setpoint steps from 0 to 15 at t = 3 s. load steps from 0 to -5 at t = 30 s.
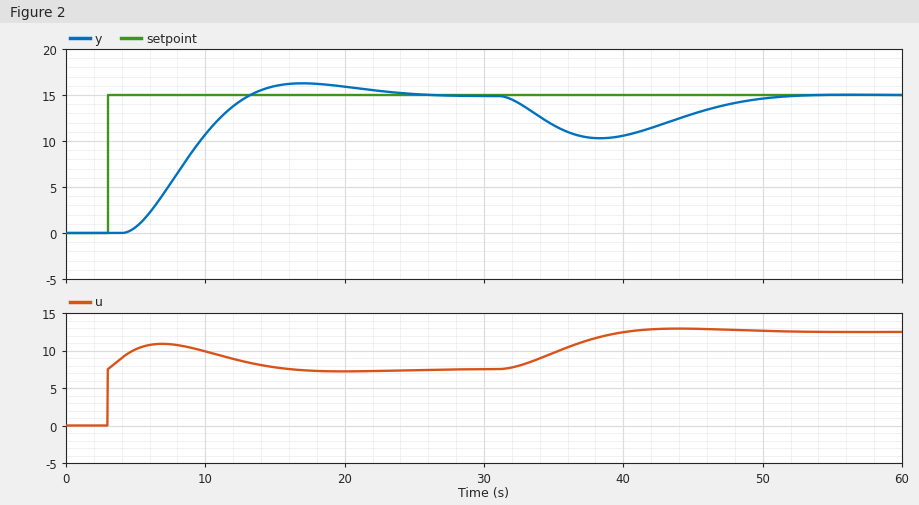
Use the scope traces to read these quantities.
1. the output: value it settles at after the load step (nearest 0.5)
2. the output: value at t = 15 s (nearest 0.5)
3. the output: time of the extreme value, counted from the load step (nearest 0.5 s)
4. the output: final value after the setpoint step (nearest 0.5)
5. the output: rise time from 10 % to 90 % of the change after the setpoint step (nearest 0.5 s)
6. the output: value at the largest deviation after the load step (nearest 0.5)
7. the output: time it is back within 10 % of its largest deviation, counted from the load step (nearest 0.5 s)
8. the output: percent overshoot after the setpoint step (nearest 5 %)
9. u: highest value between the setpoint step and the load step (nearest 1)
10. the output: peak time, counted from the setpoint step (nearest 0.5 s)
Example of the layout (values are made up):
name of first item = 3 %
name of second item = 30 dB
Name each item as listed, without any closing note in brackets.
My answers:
the output: value it settles at after the load step = 15.0
the output: value at t = 15 s = 16.0
the output: time of the extreme value, counted from the load step = 8.5 s
the output: final value after the setpoint step = 15.0
the output: rise time from 10 % to 90 % of the change after the setpoint step = 6.0 s
the output: value at the largest deviation after the load step = 10.5
the output: time it is back within 10 % of its largest deviation, counted from the load step = 19.5 s
the output: percent overshoot after the setpoint step = 10 %
u: highest value between the setpoint step and the load step = 11
the output: peak time, counted from the setpoint step = 14.0 s
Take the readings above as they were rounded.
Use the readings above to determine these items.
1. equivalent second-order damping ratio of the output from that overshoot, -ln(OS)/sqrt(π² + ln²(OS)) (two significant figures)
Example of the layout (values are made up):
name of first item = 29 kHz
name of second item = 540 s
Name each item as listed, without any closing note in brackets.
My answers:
equivalent second-order damping ratio of the output from that overshoot, -ln(OS)/sqrt(π² + ln²(OS)) = 0.59
